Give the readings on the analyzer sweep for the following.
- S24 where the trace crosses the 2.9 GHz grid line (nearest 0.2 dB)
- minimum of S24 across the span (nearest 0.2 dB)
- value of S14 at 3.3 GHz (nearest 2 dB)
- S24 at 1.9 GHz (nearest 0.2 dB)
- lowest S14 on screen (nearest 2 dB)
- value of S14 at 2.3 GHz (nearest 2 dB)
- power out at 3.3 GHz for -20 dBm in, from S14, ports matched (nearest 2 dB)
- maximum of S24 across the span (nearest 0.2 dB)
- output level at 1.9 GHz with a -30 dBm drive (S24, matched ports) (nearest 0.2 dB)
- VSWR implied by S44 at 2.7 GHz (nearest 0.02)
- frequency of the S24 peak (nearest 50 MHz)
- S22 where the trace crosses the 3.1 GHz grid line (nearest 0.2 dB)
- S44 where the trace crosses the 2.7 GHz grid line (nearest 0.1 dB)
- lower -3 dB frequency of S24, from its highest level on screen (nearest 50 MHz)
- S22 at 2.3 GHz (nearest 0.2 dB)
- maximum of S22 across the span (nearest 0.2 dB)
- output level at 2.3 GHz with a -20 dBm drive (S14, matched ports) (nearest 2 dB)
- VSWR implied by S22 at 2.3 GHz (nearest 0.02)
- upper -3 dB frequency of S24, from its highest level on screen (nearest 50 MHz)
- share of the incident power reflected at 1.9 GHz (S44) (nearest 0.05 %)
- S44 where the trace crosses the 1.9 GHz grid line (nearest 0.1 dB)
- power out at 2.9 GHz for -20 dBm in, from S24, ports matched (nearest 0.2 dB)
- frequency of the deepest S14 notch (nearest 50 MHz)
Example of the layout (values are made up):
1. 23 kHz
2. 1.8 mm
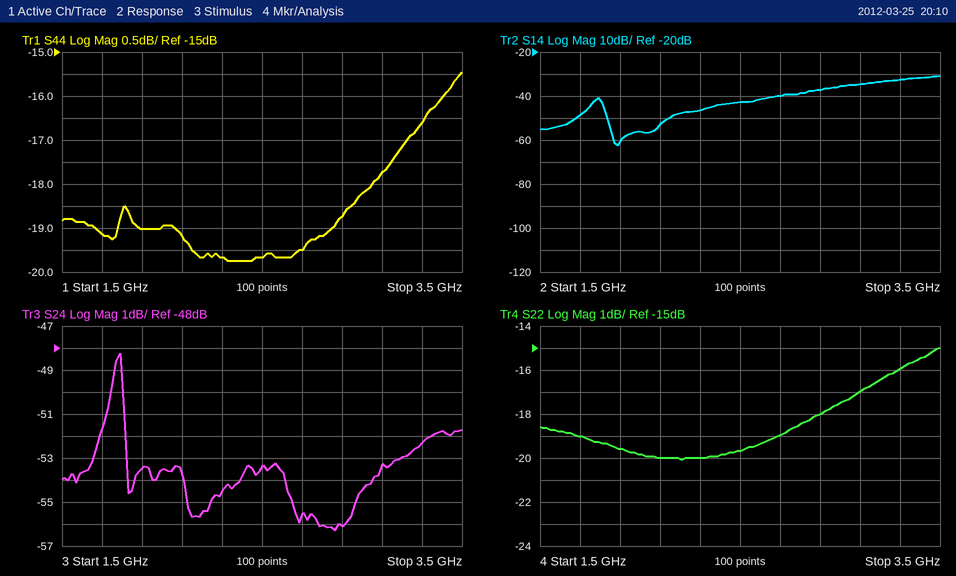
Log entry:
1. -56.0 dB
2. -56.2 dB
3. -32 dB
4. -53.4 dB
5. -62 dB
6. -46 dB
7. -52 dBm
8. -48.2 dB
9. -83.4 dBm
10. 1.24
11. 1.80 GHz
12. -17.0 dB
13. -19.5 dB
14. 1.70 GHz
15. -20.0 dB
16. -15.0 dB
17. -66 dBm
18. 1.22
19. 1.80 GHz
20. 1.25 %
21. -19.0 dB
22. -76.0 dBm
23. 1.90 GHz
